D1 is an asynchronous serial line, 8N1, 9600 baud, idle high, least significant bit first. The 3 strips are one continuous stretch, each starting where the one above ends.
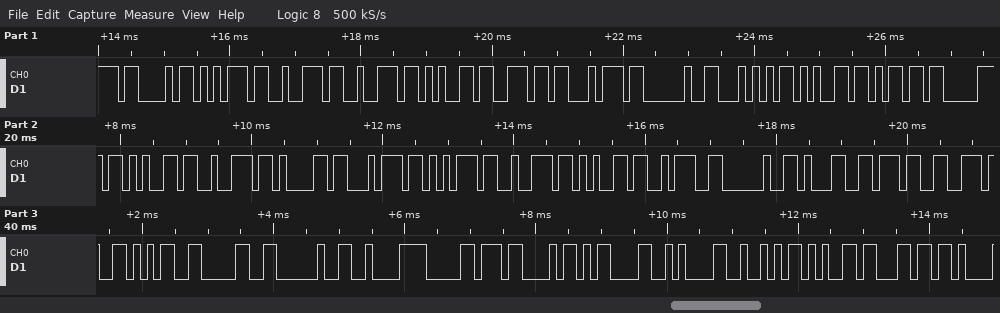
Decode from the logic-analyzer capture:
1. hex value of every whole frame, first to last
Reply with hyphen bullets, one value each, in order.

- 43 75 72 72 65 6E 74 20 54 65 6D 70 65 72 61 74 75 72 65 3A 20 31 37 2E 35 30 20 C2 B0 43 0D 0A 52 65 6C
